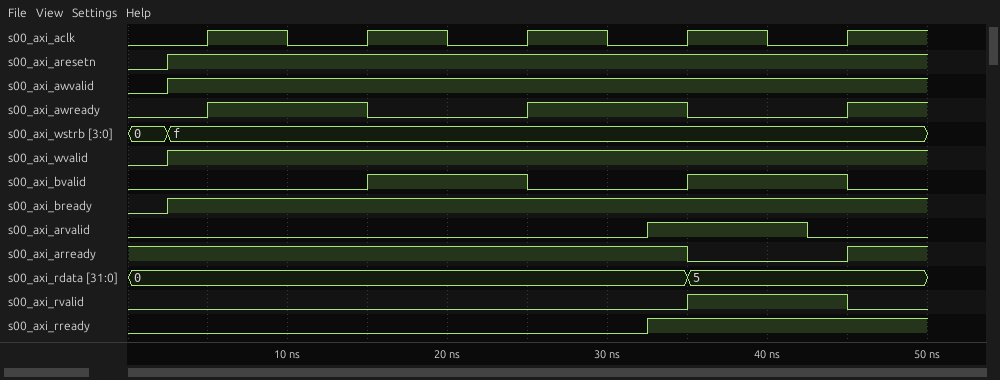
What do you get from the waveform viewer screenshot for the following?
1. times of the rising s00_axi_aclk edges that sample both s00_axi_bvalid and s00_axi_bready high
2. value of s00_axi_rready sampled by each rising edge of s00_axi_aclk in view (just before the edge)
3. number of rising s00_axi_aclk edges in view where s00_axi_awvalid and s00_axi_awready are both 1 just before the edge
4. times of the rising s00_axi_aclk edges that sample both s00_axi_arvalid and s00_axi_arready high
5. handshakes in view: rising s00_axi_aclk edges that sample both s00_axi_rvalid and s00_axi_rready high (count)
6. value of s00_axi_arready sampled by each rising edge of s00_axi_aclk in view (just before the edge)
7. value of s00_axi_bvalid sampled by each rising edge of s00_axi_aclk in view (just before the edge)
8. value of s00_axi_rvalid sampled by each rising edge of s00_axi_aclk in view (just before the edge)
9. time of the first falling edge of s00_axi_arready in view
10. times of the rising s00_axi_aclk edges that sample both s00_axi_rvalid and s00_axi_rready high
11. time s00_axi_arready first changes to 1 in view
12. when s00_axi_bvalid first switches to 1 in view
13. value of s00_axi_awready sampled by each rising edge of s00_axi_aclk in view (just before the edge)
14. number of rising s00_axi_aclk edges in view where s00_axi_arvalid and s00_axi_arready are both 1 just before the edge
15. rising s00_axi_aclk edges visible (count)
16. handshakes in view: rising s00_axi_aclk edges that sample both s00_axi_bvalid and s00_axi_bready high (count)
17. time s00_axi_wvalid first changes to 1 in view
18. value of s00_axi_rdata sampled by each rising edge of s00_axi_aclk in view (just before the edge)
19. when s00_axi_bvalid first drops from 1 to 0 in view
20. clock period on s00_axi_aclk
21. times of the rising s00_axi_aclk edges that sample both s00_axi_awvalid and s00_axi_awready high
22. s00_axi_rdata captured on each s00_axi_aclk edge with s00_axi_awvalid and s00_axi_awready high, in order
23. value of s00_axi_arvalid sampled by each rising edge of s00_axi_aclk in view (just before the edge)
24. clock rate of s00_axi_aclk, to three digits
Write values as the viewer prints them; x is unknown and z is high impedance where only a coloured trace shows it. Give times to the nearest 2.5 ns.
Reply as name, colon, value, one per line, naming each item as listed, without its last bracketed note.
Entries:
times of the rising s00_axi_aclk edges that sample both s00_axi_bvalid and s00_axi_bready high: 25 ns, 45 ns
value of s00_axi_rready sampled by each rising edge of s00_axi_aclk in view: 0 0 0 1 1
number of rising s00_axi_aclk edges in view where s00_axi_awvalid and s00_axi_awready are both 1 just before the edge: 2
times of the rising s00_axi_aclk edges that sample both s00_axi_arvalid and s00_axi_arready high: 35 ns
handshakes in view: rising s00_axi_aclk edges that sample both s00_axi_rvalid and s00_axi_rready high: 1
value of s00_axi_arready sampled by each rising edge of s00_axi_aclk in view: 1 1 1 1 0
value of s00_axi_bvalid sampled by each rising edge of s00_axi_aclk in view: 0 0 1 0 1
value of s00_axi_rvalid sampled by each rising edge of s00_axi_aclk in view: 0 0 0 0 1
time of the first falling edge of s00_axi_arready in view: 35 ns
times of the rising s00_axi_aclk edges that sample both s00_axi_rvalid and s00_axi_rready high: 45 ns
time s00_axi_arready first changes to 1 in view: 45 ns
when s00_axi_bvalid first switches to 1 in view: 15 ns
value of s00_axi_awready sampled by each rising edge of s00_axi_aclk in view: 0 1 0 1 0
number of rising s00_axi_aclk edges in view where s00_axi_arvalid and s00_axi_arready are both 1 just before the edge: 1
rising s00_axi_aclk edges visible: 5
handshakes in view: rising s00_axi_aclk edges that sample both s00_axi_bvalid and s00_axi_bready high: 2
time s00_axi_wvalid first changes to 1 in view: 2.5 ns
value of s00_axi_rdata sampled by each rising edge of s00_axi_aclk in view: 0, 0, 0, 0, 5
when s00_axi_bvalid first drops from 1 to 0 in view: 25 ns
clock period on s00_axi_aclk: 10 ns
times of the rising s00_axi_aclk edges that sample both s00_axi_awvalid and s00_axi_awready high: 15 ns, 35 ns
s00_axi_rdata captured on each s00_axi_aclk edge with s00_axi_awvalid and s00_axi_awready high, in order: 0, 0
value of s00_axi_arvalid sampled by each rising edge of s00_axi_aclk in view: 0 0 0 1 0
clock rate of s00_axi_aclk, to three digits: 100 MHz
